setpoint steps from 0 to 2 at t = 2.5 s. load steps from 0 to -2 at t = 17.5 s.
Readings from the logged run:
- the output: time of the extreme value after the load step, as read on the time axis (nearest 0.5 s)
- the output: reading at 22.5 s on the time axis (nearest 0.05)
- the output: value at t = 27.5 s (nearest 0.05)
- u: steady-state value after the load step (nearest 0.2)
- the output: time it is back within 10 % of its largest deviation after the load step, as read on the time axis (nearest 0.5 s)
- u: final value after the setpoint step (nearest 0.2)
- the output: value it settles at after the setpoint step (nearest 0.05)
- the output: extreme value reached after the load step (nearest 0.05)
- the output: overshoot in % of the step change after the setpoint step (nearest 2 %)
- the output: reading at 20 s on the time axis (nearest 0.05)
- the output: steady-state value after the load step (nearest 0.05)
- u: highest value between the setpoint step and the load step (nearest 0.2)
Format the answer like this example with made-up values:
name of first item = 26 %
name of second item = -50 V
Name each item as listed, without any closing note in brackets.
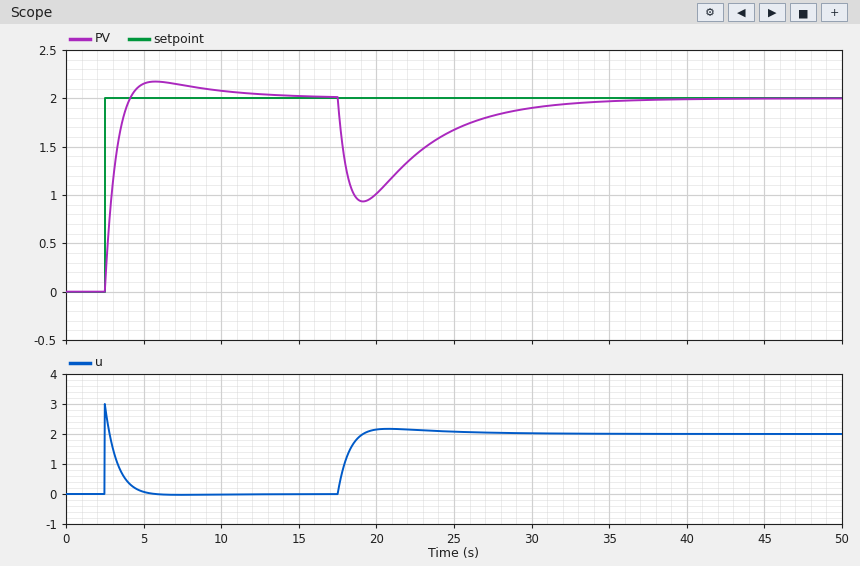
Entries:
the output: time of the extreme value after the load step, as read on the time axis = 19.0 s
the output: reading at 22.5 s on the time axis = 1.40
the output: value at t = 27.5 s = 1.80
u: steady-state value after the load step = 2.0
the output: time it is back within 10 % of its largest deviation after the load step, as read on the time axis = 29.5 s
u: final value after the setpoint step = 0.0
the output: value it settles at after the setpoint step = 2.00
the output: extreme value reached after the load step = 0.95
the output: overshoot in % of the step change after the setpoint step = 8 %
the output: reading at 20 s on the time axis = 1.00
the output: steady-state value after the load step = 2.00
u: highest value between the setpoint step and the load step = 3.0
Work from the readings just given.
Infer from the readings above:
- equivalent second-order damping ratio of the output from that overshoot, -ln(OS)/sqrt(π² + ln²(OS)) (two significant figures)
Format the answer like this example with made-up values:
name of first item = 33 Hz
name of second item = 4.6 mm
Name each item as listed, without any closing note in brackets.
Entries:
equivalent second-order damping ratio of the output from that overshoot, -ln(OS)/sqrt(π² + ln²(OS)) = 0.63
